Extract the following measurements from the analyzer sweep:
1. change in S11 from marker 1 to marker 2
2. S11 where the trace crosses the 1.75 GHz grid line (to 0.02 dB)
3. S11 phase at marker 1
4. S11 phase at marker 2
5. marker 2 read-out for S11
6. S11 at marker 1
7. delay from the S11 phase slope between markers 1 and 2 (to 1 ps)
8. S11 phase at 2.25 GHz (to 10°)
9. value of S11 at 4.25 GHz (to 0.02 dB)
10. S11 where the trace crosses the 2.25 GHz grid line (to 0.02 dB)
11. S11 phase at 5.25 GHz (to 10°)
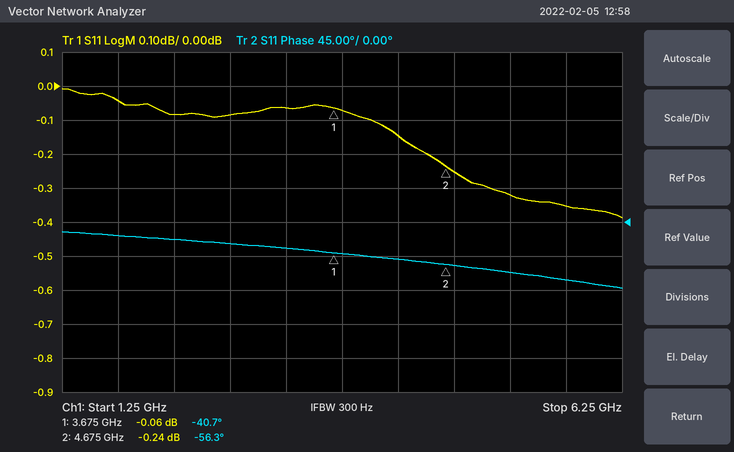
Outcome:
-0.18 dB
-0.04 dB
-40.7°
-56.3°
-0.24 dB
-0.06 dB
43 ps
-20°
-0.14 dB
-0.08 dB
-70°
